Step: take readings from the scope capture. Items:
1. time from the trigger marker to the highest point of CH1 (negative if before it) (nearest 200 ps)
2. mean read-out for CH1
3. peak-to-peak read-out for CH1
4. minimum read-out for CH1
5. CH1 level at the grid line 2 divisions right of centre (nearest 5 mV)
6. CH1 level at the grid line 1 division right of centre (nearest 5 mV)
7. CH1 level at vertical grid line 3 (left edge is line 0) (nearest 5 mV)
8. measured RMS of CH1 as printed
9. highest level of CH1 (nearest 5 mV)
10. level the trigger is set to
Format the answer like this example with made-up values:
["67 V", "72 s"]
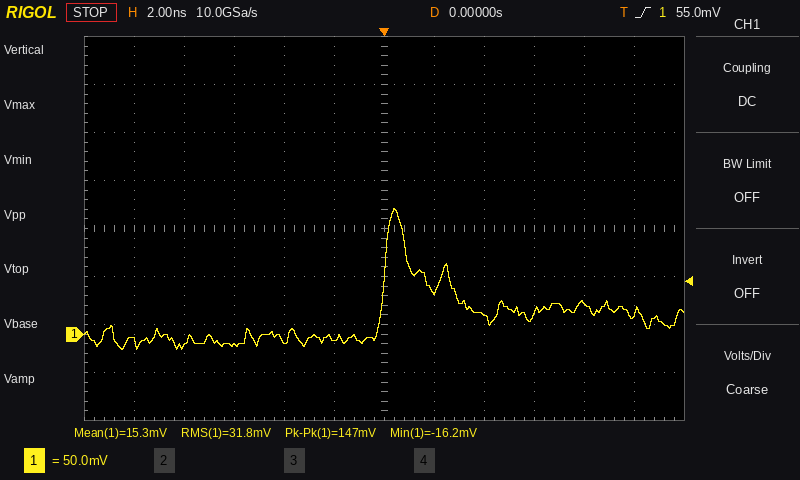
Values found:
["+400 ps", "15.3 mV", "147 mV", "-16.2 mV", "20 mV", "45 mV", "-10 mV", "31.8 mV", "130 mV", "55.0 mV"]
